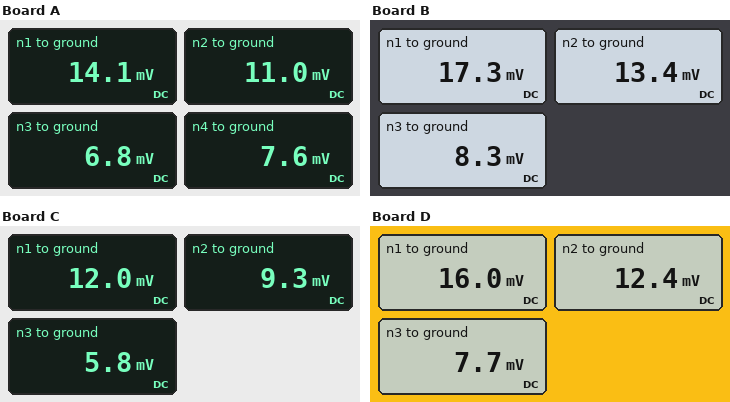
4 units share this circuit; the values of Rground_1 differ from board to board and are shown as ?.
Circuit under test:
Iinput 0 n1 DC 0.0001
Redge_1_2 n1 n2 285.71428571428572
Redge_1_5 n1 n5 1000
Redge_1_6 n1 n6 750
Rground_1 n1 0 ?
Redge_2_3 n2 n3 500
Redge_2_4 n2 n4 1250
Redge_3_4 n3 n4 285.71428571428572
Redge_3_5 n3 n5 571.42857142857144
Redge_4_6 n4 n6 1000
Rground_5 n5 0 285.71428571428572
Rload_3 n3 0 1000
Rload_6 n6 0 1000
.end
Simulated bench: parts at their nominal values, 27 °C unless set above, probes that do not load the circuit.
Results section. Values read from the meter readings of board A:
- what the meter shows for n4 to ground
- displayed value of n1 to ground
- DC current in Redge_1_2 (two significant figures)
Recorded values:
7.6 mV
14.1 mV
11 µA
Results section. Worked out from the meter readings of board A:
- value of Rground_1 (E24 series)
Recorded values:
200 Ω
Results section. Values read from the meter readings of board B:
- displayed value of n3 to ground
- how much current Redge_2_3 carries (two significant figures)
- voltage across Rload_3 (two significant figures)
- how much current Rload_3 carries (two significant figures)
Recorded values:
8.3 mV
10 µA
8.3 mV
8.3 µA
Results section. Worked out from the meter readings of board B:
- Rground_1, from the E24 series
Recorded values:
270 Ω
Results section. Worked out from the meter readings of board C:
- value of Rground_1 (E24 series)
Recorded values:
160 Ω
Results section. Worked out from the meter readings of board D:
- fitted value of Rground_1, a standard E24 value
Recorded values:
240 Ω
